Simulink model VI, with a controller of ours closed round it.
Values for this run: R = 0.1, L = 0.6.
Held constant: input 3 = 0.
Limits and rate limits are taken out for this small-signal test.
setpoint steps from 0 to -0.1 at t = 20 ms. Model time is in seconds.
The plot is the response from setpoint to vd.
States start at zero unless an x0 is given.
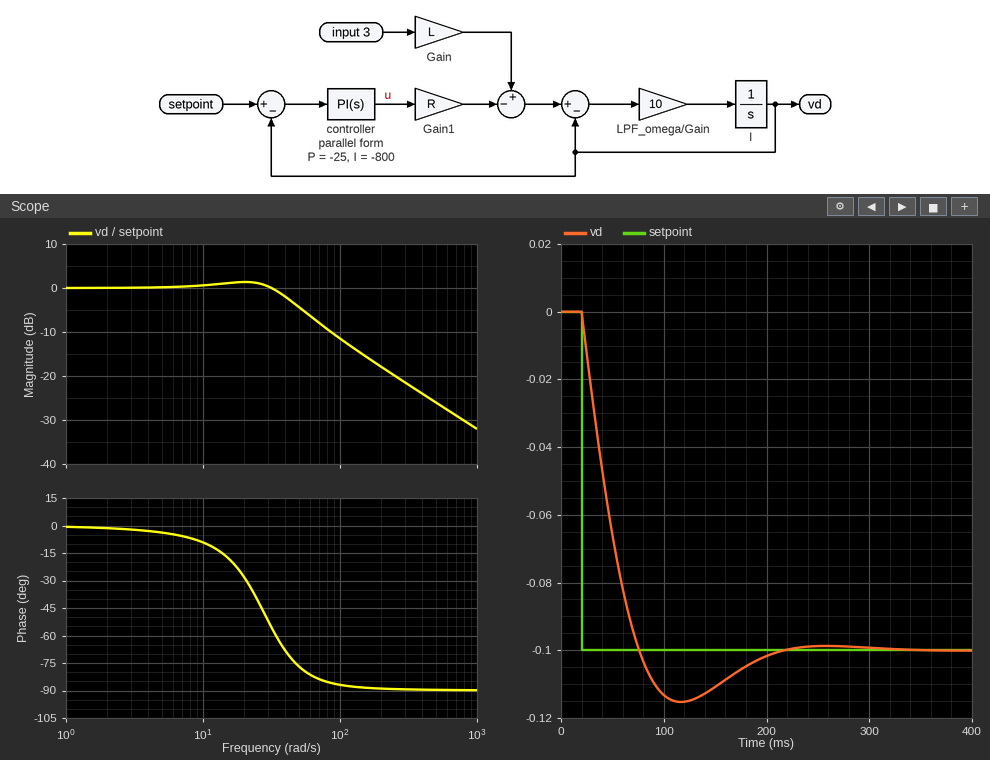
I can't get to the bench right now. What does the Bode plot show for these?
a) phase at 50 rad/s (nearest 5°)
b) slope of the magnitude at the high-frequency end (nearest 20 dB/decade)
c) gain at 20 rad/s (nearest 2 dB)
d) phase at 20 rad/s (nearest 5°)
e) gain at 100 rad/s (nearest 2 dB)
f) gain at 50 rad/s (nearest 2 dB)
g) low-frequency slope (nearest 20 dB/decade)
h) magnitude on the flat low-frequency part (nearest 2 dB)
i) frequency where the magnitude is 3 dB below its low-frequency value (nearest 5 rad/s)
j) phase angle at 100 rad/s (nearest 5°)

-75°
-20 dB/decade
2 dB
-30°
-12 dB
-4 dB
0 dB/decade
0 dB
45 rad/s
-85°
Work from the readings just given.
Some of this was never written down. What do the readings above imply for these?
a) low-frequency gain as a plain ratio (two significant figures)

1.0
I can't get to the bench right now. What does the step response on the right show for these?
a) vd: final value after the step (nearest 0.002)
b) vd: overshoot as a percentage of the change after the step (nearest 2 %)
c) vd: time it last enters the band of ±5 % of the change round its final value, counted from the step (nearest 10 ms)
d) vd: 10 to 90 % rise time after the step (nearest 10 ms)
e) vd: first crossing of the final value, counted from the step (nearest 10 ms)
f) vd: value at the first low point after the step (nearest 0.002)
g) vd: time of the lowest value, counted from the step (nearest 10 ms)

-0.100
16 %
160 ms
40 ms
60 ms
-0.116
100 ms
